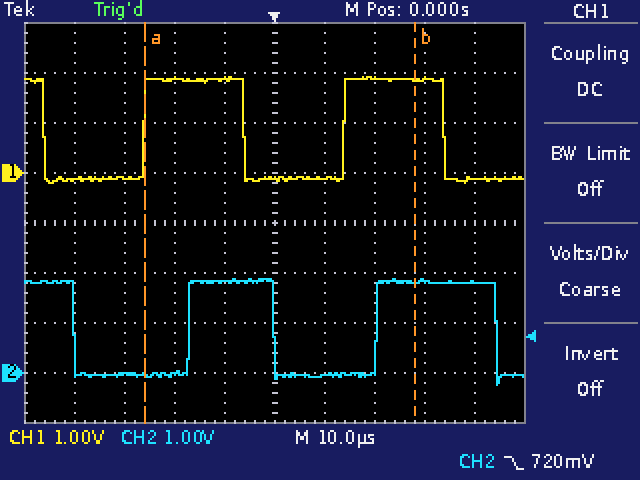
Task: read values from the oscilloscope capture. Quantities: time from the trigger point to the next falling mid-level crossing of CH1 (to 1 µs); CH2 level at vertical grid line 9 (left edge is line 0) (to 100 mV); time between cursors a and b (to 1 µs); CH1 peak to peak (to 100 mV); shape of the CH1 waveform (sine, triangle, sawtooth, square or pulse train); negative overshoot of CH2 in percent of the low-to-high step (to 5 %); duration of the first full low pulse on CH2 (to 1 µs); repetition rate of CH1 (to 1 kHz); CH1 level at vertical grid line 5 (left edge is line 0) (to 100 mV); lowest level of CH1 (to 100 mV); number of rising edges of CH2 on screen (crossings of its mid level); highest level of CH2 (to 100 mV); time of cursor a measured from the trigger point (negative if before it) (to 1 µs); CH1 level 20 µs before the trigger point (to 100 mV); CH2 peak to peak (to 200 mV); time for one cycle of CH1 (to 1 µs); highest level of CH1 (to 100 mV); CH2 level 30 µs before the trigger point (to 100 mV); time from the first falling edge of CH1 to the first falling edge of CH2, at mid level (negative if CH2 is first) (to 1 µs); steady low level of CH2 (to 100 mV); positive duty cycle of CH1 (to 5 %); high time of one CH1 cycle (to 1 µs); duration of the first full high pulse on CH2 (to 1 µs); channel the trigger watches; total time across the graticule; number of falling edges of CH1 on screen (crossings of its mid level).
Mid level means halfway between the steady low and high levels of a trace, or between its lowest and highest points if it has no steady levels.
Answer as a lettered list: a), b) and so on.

a) 34 µs
b) 1.8 V
c) 54 µs
d) 2.1 V
e) square
f) 10 %
g) 23 µs
h) 25 kHz
i) -100 mV
j) -200 mV
k) 2
l) 1.9 V
m) -26 µs
n) 1.9 V
o) 2.2 V
p) 40 µs
q) 1.9 V
r) 0.0 V
s) +6 µs
t) 0.0 V
u) 50 %
v) 20 µs
w) 17 µs
x) CH2
y) 100 µs
z) 3
